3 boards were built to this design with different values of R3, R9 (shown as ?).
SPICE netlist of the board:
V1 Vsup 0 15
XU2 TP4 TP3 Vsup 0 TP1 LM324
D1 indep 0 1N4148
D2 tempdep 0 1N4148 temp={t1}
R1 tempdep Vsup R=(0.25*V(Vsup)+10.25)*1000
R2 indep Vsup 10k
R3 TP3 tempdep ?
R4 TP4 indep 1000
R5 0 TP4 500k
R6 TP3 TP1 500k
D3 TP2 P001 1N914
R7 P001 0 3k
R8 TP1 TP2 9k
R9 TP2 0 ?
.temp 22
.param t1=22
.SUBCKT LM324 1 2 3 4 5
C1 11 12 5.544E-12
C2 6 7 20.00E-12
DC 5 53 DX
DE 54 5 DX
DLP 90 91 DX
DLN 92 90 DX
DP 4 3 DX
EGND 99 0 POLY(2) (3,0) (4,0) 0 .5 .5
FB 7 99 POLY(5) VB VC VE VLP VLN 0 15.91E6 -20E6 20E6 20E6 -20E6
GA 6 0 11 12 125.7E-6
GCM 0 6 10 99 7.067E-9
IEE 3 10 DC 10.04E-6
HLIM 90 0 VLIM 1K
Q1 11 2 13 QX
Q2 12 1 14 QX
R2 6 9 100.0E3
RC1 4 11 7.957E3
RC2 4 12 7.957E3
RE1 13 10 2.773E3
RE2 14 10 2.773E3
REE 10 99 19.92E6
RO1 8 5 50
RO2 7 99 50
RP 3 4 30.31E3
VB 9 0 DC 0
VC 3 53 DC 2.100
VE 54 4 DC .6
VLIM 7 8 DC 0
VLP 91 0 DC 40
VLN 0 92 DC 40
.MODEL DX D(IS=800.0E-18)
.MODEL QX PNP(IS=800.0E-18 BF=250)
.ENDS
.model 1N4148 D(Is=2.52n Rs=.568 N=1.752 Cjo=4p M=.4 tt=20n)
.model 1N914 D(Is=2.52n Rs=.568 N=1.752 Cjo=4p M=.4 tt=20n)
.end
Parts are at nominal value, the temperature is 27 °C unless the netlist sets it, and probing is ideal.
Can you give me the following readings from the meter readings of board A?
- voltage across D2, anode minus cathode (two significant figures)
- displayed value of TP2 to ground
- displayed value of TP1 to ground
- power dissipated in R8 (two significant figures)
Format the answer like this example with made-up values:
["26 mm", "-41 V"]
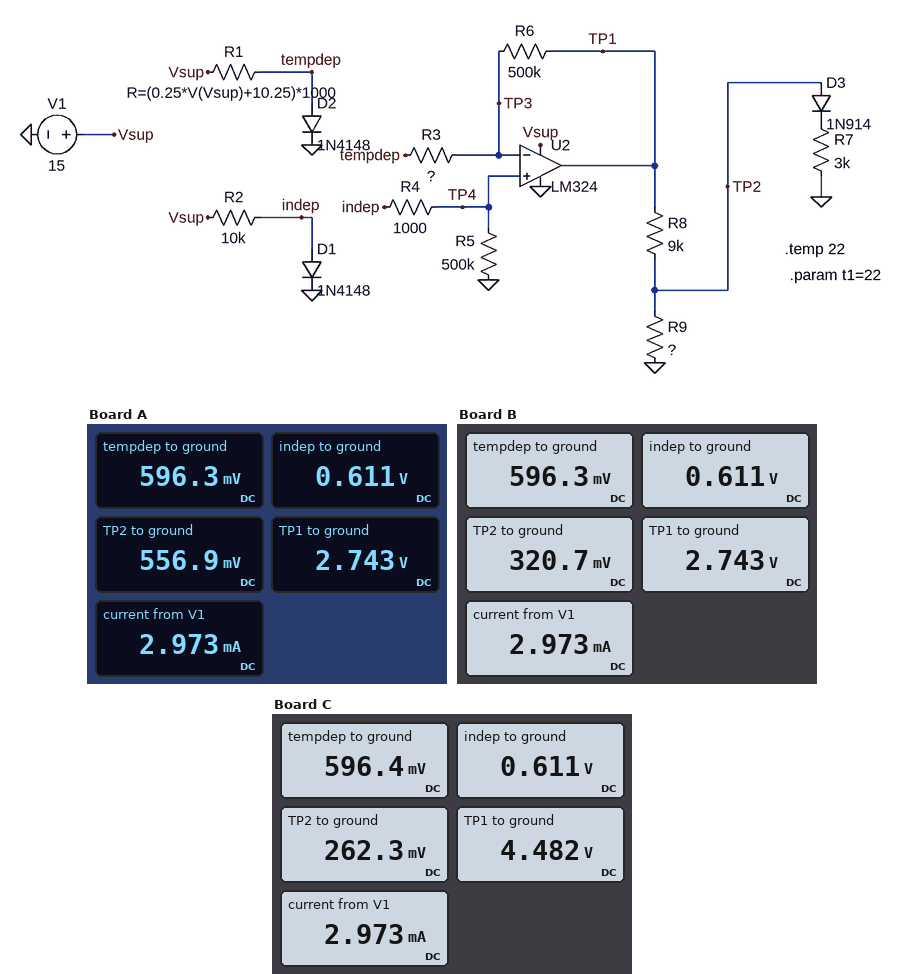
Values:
["600 mV", "556.9 mV", "2.743 V", "530 µW"]
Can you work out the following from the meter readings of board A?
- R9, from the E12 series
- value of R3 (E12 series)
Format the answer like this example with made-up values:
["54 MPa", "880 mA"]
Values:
["2.7 kΩ", "3.3 kΩ"]
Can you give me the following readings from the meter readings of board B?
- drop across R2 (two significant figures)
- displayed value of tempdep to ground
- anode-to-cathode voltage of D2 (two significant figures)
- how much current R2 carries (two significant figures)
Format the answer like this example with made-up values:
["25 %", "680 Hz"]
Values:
["14 V", "596.3 mV", "600 mV", "1.4 mA"]
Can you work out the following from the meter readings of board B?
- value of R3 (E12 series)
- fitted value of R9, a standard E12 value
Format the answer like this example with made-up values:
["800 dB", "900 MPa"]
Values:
["3.3 kΩ", "1.2 kΩ"]
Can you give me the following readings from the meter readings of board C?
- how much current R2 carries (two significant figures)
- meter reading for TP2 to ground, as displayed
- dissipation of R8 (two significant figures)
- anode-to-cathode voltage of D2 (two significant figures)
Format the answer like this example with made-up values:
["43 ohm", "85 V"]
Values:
["1.4 mA", "262.3 mV", "2.0 mW", "600 mV"]
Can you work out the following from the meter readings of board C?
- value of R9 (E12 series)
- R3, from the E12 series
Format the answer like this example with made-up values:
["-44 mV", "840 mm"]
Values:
["560 Ω", "1.8 kΩ"]
